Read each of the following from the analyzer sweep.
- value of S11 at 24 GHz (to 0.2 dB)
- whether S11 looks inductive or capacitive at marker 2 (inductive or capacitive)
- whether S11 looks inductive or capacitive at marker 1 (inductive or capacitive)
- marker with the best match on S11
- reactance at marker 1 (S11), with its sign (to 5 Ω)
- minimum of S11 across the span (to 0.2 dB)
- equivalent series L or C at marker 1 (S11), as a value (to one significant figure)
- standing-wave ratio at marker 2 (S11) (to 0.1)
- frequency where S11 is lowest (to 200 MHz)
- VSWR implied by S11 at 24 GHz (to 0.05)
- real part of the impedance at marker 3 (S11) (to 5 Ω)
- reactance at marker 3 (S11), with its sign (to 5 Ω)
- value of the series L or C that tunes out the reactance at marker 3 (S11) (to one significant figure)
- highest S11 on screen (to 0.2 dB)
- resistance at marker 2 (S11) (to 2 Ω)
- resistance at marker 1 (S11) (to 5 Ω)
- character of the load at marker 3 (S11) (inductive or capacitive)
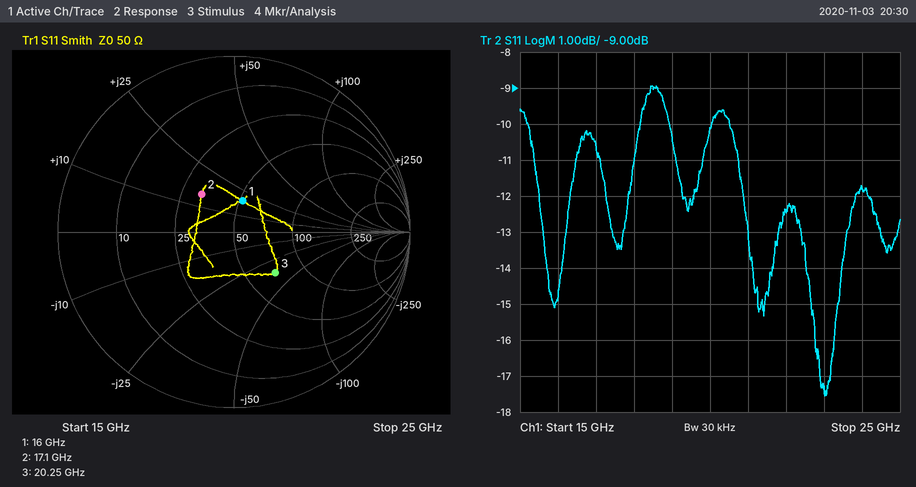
-11.8 dB
inductive
inductive
marker 1
+20 Ω
-17.6 dB
200 pH
1.8
23.0 GHz
1.70
70 Ω
-35 Ω
300 pH
-9.0 dB
32 Ω
50 Ω
capacitive
